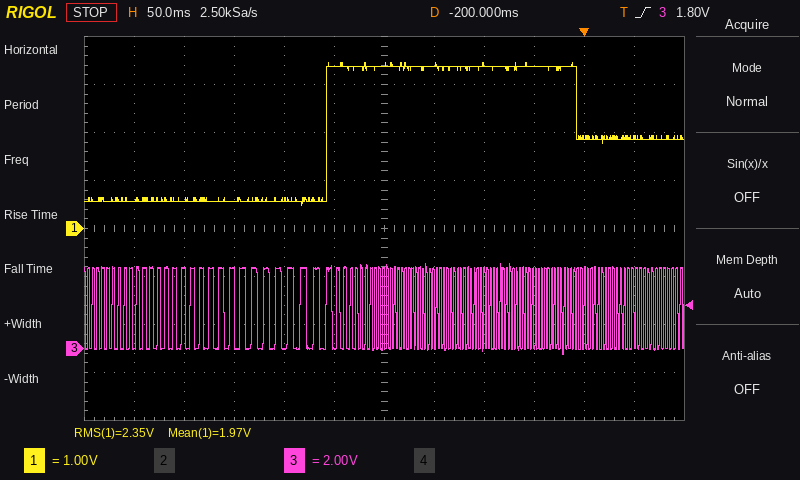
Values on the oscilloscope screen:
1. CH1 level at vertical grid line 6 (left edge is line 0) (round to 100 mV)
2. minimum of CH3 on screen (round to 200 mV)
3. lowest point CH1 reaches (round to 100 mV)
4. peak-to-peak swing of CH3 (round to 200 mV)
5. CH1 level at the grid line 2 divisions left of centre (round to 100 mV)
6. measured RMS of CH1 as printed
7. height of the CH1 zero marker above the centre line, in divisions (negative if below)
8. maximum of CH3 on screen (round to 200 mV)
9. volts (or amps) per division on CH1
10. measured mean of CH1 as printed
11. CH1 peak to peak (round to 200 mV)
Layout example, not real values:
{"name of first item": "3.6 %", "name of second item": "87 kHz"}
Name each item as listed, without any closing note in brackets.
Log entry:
{"CH1 level at vertical grid line 6 (left edge is line 0)": "3.4 V", "minimum of CH3 on screen": "-200 mV", "lowest point CH1 reaches": "500 mV", "peak-to-peak swing of CH3": "3.8 V", "CH1 level at the grid line 2 divisions left of centre": "600 mV", "measured RMS of CH1 as printed": "2.35 V", "height of the CH1 zero marker above the centre line, in divisions": "0.0 div", "maximum of CH3 on screen": "3.6 V", "volts (or amps) per division on CH1": "1 V", "measured mean of CH1 as printed": "1.97 V", "CH1 peak to peak": "3.0 V"}
